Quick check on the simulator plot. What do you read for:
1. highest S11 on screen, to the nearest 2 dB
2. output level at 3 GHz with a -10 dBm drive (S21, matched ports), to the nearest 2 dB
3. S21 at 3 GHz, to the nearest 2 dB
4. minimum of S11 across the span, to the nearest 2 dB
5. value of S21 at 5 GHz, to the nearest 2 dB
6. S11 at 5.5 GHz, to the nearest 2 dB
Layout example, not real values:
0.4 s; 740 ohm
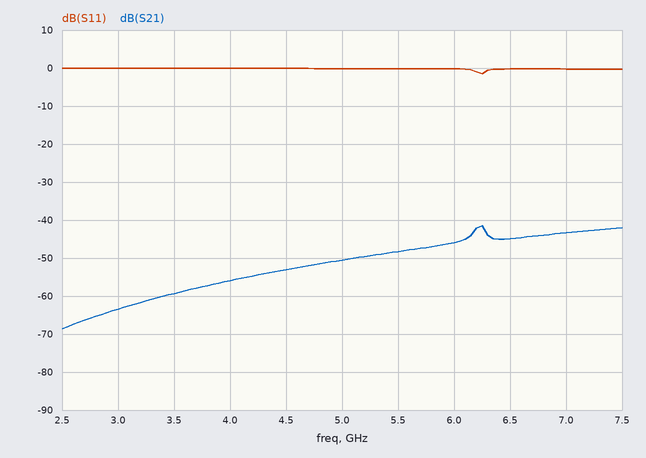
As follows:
0 dB; -74 dBm; -64 dB; -2 dB; -50 dB; 0 dB
